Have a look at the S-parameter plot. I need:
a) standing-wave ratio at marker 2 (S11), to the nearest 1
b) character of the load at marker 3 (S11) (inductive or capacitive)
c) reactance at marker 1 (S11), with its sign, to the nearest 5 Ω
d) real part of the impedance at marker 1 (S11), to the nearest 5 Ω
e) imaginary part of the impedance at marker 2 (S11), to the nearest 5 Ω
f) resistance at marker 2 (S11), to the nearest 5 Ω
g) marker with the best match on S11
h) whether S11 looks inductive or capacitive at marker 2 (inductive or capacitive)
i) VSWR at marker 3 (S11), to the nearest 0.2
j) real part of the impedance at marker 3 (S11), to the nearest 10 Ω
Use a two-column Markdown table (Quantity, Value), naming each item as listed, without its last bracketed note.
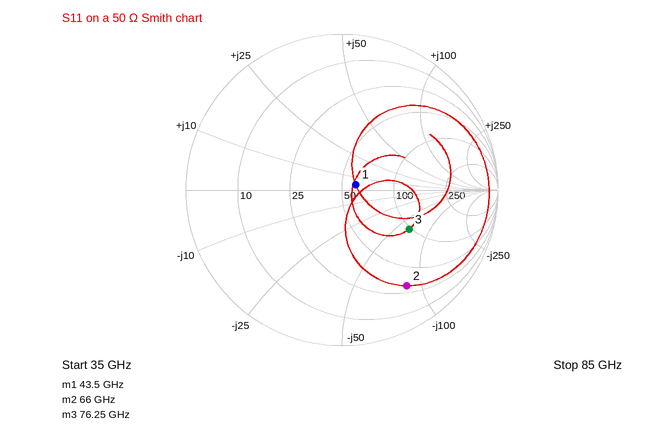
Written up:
| Quantity | Value |
|---|---|
| standing-wave ratio at marker 2 (S11), to the nearest 1 | 7 |
| character of the load at marker 3 (S11) | capacitive |
| reactance at marker 1 (S11), with its sign, to the nearest 5 Ω | +5 Ω |
| real part of the impedance at marker 1 (S11), to the nearest 5 Ω | 60 Ω |
| imaginary part of the impedance at marker 2 (S11), to the nearest 5 Ω | -85 Ω |
| resistance at marker 2 (S11), to the nearest 5 Ω | 30 Ω |
| marker with the best match on S11 | marker 1 |
| whether S11 looks inductive or capacitive at marker 2 | capacitive |
| VSWR at marker 3 (S11), to the nearest 0.2 | 3.0 |
| real part of the impedance at marker 3 (S11), to the nearest 10 Ω | 100 Ω |
